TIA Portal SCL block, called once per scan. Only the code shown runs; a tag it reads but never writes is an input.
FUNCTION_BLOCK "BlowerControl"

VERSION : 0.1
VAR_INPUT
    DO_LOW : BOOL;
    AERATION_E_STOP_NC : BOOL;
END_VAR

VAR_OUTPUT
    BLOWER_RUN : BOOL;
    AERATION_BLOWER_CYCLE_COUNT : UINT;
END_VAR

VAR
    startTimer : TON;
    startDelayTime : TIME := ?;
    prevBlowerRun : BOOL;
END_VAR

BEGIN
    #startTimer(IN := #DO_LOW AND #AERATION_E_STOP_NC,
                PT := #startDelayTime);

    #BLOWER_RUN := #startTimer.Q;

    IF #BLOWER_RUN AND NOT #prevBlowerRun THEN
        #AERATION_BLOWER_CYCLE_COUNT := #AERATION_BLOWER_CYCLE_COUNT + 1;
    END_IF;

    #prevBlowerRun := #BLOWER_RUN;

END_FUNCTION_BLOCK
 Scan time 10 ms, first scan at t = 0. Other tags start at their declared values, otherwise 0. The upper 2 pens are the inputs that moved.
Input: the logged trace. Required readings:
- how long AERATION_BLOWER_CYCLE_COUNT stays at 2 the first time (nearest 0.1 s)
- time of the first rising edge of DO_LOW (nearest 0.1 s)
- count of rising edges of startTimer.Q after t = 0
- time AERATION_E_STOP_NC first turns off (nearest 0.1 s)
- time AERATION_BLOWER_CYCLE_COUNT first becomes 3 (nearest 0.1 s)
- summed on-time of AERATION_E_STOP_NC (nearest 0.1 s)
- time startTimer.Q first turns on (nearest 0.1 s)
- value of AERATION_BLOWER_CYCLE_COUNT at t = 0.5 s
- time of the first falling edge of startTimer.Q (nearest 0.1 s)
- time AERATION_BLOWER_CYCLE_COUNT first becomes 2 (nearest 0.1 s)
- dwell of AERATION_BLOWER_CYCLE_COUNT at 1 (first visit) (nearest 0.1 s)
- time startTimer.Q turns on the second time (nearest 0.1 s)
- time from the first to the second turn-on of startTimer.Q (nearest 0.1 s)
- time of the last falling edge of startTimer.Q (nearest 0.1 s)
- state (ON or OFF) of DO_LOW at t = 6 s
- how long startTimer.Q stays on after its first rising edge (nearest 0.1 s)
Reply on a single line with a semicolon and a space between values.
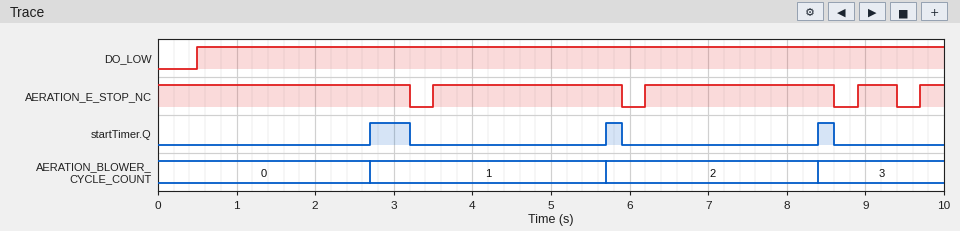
2.7 s; 0.5 s; 3; 3.2 s; 8.4 s; 8.8 s; 2.7 s; 0; 3.2 s; 5.7 s; 3.0 s; 5.7 s; 3.0 s; 8.6 s; ON; 0.5 s
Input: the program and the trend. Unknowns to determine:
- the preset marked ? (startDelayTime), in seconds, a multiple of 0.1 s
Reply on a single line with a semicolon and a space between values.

2.2 s
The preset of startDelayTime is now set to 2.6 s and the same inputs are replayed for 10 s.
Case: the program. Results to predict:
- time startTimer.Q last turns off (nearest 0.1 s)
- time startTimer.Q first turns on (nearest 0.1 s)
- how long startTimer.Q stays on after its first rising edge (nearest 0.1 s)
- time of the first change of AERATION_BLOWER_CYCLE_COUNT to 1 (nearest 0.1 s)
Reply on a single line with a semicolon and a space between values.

3.2 s; 3.1 s; 0.1 s; 3.1 s
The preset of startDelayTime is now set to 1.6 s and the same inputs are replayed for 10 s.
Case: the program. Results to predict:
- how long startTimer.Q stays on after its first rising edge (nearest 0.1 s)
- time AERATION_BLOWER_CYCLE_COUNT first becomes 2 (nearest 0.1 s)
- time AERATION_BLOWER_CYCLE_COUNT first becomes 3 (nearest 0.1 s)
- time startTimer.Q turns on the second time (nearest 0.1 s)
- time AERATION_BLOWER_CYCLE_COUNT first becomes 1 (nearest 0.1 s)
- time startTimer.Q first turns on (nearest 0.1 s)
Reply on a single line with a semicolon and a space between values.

1.1 s; 5.1 s; 7.8 s; 5.1 s; 2.1 s; 2.1 s
